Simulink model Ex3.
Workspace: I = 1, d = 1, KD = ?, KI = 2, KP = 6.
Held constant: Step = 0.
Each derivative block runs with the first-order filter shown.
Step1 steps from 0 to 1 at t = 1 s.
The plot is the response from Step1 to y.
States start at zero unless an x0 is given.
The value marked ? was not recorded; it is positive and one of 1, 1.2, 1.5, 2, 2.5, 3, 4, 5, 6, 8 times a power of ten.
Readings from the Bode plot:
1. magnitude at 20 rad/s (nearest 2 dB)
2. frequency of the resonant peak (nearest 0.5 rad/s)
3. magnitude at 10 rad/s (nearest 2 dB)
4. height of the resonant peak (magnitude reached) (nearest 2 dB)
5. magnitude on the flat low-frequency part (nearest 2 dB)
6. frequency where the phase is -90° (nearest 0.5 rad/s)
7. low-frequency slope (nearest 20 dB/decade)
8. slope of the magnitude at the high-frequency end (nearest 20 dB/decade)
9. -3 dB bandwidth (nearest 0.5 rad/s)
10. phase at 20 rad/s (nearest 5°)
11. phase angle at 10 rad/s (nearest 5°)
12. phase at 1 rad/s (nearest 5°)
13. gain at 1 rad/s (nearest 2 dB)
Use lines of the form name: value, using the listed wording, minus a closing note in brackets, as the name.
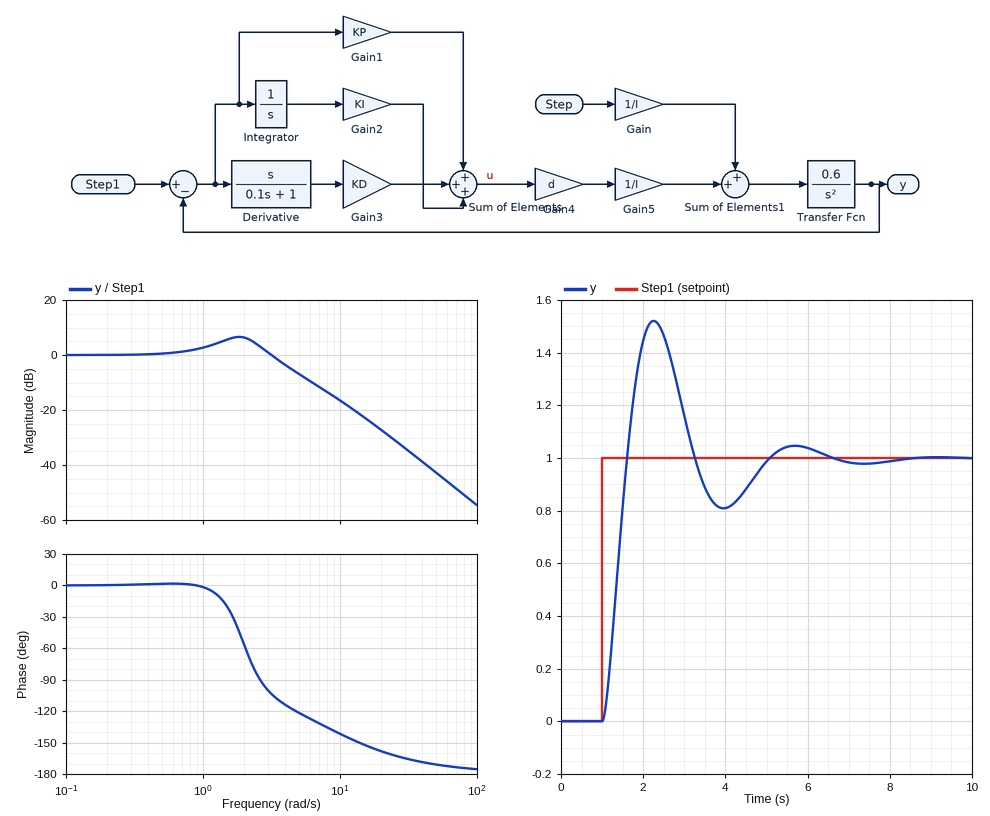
magnitude at 20 rad/s: -28 dB
frequency of the resonant peak: 2.0 rad/s
magnitude at 10 rad/s: -16 dB
height of the resonant peak (magnitude reached): 6 dB
magnitude on the flat low-frequency part: 0 dB
frequency where the phase is -90°: 2.5 rad/s
low-frequency slope: 0 dB/decade
slope of the magnitude at the high-frequency end: -40 dB/decade
-3 dB bandwidth: 4.0 rad/s
phase at 20 rad/s: -160°
phase angle at 10 rad/s: -140°
phase at 1 rad/s: 0°
gain at 1 rad/s: 2 dB
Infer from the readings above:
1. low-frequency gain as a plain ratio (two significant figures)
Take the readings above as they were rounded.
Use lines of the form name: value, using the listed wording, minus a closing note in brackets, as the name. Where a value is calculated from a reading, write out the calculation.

low-frequency gain as a plain ratio: 10^(0 / 20) = 1.0
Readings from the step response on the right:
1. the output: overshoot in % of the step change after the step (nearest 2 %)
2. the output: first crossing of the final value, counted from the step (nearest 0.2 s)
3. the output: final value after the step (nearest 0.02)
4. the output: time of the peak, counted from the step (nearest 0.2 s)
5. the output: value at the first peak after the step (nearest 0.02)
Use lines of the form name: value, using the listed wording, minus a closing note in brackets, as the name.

the output: overshoot in % of the step change after the step: 52 %
the output: first crossing of the final value, counted from the step: 0.6 s
the output: final value after the step: 1.00
the output: time of the peak, counted from the step: 1.2 s
the output: value at the first peak after the step: 1.52
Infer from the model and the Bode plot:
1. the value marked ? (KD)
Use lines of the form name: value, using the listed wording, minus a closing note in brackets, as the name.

the value marked ?: 2.5
